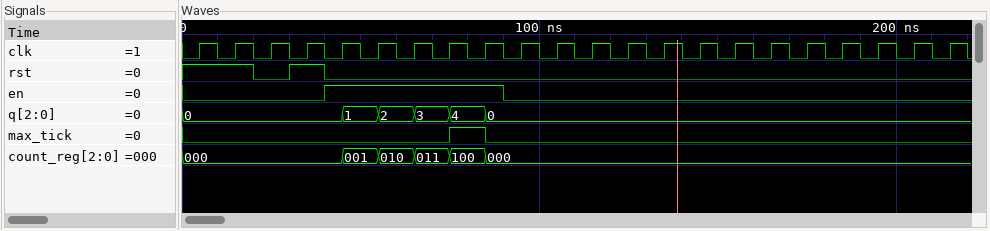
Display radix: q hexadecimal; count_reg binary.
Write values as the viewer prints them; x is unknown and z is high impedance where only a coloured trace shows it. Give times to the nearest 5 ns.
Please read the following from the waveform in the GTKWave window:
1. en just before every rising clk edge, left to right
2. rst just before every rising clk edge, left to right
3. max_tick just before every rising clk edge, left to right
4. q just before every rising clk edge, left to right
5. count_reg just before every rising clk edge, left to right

0 0 0 0 1 1 1 1 1 0 0 0 0 0 0 0 0 0 0 0 0 0
1 1 0 1 0 0 0 0 0 0 0 0 0 0 0 0 0 0 0 0 0 0
0 0 0 0 0 0 0 0 1 0 0 0 0 0 0 0 0 0 0 0 0 0
0, 0, 0, 0, 0, 1, 2, 3, 4, 0, 0, 0, 0, 0, 0, 0, 0, 0, 0, 0, 0, 0
000, 000, 000, 000, 000, 001, 010, 011, 100, 000, 000, 000, 000, 000, 000, 000, 000, 000, 000, 000, 000, 000
